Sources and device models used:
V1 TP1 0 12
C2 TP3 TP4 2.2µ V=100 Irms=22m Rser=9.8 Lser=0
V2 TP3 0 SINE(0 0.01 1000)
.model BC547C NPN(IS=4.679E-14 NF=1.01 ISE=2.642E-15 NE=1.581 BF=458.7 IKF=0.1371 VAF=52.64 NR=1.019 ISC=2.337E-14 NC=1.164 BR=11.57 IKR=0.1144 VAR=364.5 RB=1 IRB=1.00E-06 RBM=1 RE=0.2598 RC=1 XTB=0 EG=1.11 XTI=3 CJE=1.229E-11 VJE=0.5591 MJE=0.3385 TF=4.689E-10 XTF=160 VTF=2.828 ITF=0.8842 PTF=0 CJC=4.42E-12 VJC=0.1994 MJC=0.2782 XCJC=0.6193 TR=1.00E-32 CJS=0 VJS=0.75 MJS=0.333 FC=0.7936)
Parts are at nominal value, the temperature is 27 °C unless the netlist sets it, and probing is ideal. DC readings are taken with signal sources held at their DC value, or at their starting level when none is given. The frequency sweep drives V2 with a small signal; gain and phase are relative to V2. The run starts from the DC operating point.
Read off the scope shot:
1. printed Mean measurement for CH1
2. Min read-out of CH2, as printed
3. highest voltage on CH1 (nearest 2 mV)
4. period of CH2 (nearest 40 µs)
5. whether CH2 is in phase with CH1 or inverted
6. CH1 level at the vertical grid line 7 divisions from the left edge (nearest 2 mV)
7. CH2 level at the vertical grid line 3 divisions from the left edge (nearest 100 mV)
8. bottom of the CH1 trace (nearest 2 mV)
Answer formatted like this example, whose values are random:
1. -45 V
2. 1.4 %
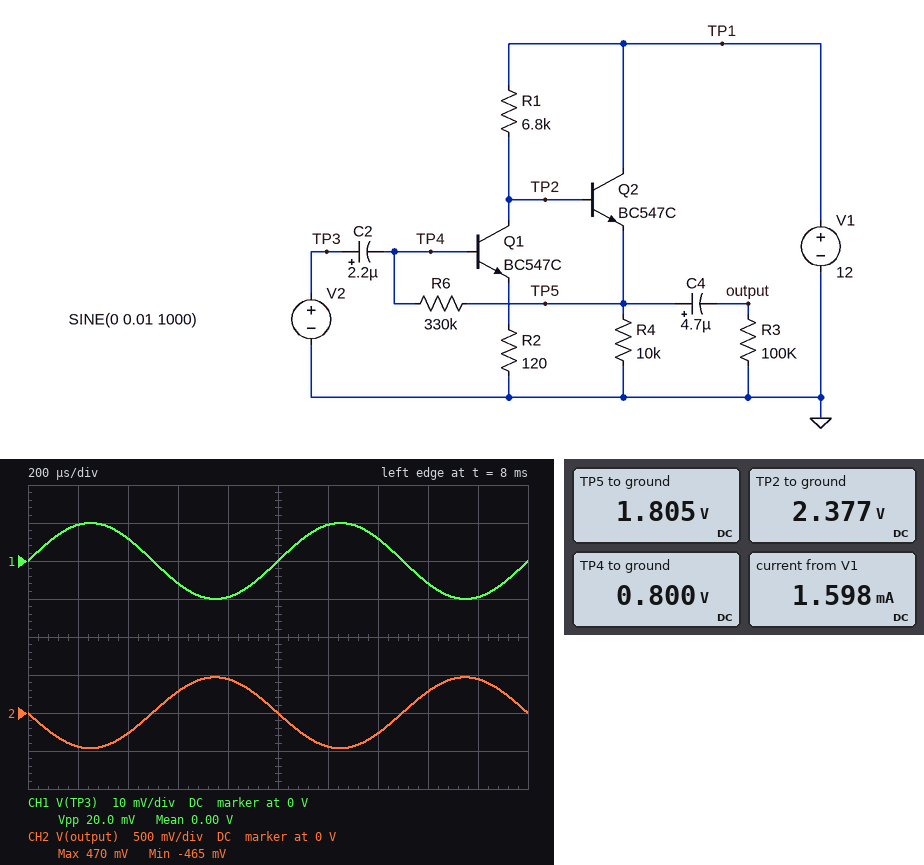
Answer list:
1. 0.00 V
2. -465 mV
3. 10 mV
4. 1.00 ms
5. inverted
6. 6 mV
7. 300 mV
8. -10 mV
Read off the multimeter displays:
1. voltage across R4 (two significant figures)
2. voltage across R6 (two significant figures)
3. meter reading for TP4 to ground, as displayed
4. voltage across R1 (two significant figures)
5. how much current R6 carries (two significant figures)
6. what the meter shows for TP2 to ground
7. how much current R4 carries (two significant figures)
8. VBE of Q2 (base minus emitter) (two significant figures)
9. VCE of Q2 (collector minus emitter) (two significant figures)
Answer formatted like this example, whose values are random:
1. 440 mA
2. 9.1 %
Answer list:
1. 1.8 V
2. 1.0 V
3. 0.800 V
4. 9.6 V
5. 3.0 µA
6. 2.377 V
7. 180 µA
8. 570 mV
9. 10 V
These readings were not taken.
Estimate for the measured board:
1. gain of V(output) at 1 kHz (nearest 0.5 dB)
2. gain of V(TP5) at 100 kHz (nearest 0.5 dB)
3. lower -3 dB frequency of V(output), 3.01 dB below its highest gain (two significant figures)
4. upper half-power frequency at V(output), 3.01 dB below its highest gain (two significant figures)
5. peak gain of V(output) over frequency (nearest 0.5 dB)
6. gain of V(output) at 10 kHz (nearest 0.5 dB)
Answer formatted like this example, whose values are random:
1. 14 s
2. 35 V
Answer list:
1. 33.5 dB
2. 33.5 dB
3. 12 Hz
4. 5.1 MHz
5. 33.5 dB
6. 33.5 dB
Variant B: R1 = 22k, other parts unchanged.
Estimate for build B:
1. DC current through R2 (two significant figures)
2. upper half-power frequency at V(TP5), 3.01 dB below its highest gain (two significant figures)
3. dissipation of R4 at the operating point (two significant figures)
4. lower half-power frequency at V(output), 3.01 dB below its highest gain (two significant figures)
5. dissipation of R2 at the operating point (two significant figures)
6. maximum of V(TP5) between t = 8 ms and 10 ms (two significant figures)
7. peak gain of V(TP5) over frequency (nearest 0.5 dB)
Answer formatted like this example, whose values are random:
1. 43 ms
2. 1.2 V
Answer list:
1. 480 µA
2. 1.5 MHz
3. 100 µW
4. 26 Hz
5. 27 µW
6. 2.1 V
7. 41.0 dB
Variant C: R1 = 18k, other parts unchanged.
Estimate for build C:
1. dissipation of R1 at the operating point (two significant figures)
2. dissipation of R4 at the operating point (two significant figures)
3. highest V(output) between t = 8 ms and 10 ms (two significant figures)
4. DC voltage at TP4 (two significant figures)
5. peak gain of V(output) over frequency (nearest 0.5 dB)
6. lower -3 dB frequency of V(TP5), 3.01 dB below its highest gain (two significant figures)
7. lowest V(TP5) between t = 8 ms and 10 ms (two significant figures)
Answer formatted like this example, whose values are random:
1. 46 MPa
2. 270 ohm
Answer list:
1. 6.0 mW
2. 120 µW
3. 990 mV
4. 680 mV
5. 40.0 dB
6. 23 Hz
7. 150 mV
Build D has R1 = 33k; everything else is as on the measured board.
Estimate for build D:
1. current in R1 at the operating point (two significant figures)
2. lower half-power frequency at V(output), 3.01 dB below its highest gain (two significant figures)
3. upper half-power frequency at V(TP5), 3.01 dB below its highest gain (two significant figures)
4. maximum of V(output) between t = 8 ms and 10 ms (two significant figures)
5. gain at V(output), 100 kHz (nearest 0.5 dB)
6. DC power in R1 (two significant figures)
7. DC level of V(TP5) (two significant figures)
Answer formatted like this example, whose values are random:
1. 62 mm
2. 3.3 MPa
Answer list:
1. 320 µA
2. 33 Hz
3. 960 kHz
4. 1.4 V
5. 43.0 dB
6. 3.4 mW
7. 860 mV
